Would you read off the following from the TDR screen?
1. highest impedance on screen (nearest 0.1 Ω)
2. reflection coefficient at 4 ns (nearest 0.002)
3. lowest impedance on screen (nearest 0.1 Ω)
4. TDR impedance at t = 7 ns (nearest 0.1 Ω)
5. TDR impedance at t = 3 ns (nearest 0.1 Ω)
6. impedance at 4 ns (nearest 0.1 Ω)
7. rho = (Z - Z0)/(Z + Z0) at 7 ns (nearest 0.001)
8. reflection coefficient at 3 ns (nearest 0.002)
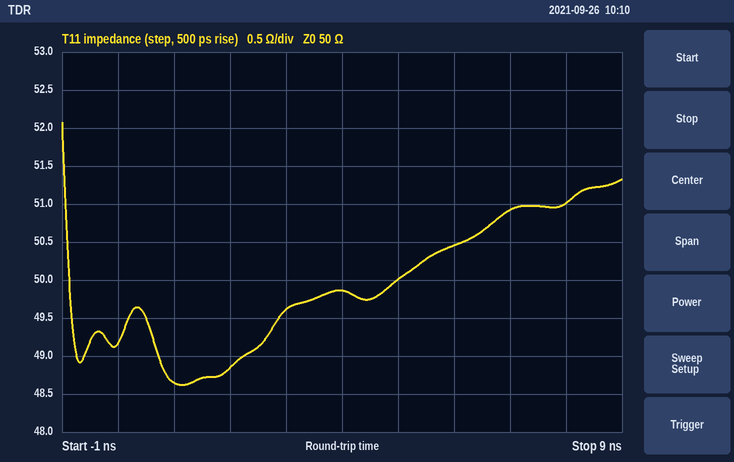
52.1 Ω
-0.002
48.6 Ω
50.9 Ω
49.6 Ω
49.9 Ω
+0.009
-0.004
